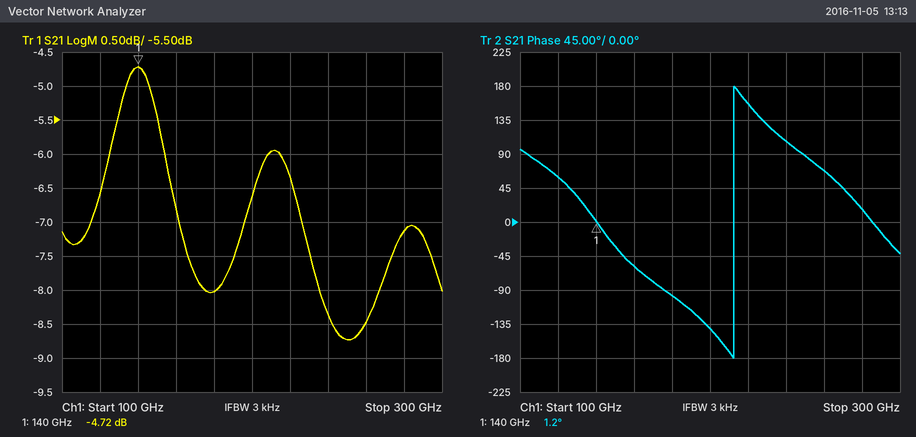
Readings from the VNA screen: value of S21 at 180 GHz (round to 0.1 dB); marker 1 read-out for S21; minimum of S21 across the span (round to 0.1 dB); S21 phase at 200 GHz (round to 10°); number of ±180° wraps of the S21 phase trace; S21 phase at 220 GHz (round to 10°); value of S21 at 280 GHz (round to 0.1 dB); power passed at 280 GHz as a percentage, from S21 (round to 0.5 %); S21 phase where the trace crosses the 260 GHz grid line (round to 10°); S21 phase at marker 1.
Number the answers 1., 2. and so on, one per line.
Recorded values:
1. -8.0 dB
2. -4.72 dB
3. -8.7 dB
4. -140°
5. 1
6. 160°
7. -7.1 dB
8. 19.5 %
9. 70°
10. 1.2°
